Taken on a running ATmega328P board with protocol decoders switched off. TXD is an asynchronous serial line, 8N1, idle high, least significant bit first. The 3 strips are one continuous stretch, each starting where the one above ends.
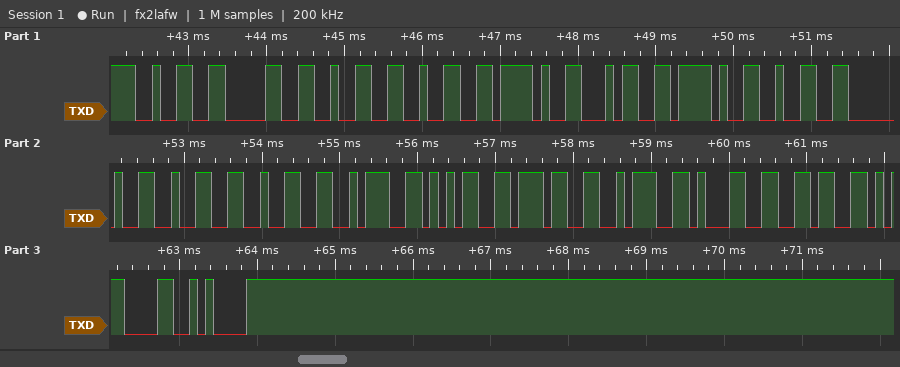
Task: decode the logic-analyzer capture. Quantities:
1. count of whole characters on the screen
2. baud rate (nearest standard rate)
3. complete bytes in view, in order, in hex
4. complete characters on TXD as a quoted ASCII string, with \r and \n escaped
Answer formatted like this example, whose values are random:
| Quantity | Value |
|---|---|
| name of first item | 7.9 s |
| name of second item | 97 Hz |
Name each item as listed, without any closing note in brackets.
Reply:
| Quantity | Value |
|---|---|
| count of whole characters on the screen | 19 |
| baud rate | 9600 baud |
| complete bytes in view, in order, in hex | 32 30 32 32 2F 34 2F 32 20 32 32 3A 35 37 3A 31 36 0D 0A |
| complete characters on TXD as a quoted ASCII string, with \r and \n escaped | "2022/4/2 22:57:16\r\n" |
